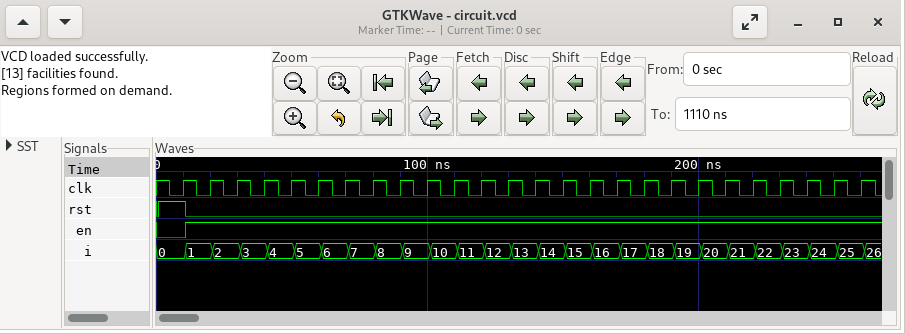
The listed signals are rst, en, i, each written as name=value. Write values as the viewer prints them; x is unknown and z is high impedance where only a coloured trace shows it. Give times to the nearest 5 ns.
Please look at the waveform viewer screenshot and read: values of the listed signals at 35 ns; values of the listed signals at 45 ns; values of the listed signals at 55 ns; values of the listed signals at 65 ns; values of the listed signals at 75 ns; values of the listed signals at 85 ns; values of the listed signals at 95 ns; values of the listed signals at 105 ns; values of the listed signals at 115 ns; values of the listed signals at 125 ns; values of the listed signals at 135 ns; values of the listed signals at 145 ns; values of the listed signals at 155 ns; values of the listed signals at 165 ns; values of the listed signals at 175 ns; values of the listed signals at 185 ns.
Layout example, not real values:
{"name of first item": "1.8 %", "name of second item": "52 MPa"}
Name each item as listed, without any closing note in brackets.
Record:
{"values of the listed signals at 35 ns": "rst=0, en=1, i=3", "values of the listed signals at 45 ns": "rst=0, en=1, i=4", "values of the listed signals at 55 ns": "rst=0, en=1, i=5", "values of the listed signals at 65 ns": "rst=0, en=1, i=6", "values of the listed signals at 75 ns": "rst=0, en=1, i=7", "values of the listed signals at 85 ns": "rst=0, en=1, i=8", "values of the listed signals at 95 ns": "rst=0, en=1, i=9", "values of the listed signals at 105 ns": "rst=0, en=1, i=10", "values of the listed signals at 115 ns": "rst=0, en=1, i=11", "values of the listed signals at 125 ns": "rst=0, en=1, i=12", "values of the listed signals at 135 ns": "rst=0, en=1, i=13", "values of the listed signals at 145 ns": "rst=0, en=1, i=14", "values of the listed signals at 155 ns": "rst=0, en=1, i=15", "values of the listed signals at 165 ns": "rst=0, en=1, i=16", "values of the listed signals at 175 ns": "rst=0, en=1, i=17", "values of the listed signals at 185 ns": "rst=0, en=1, i=18"}
